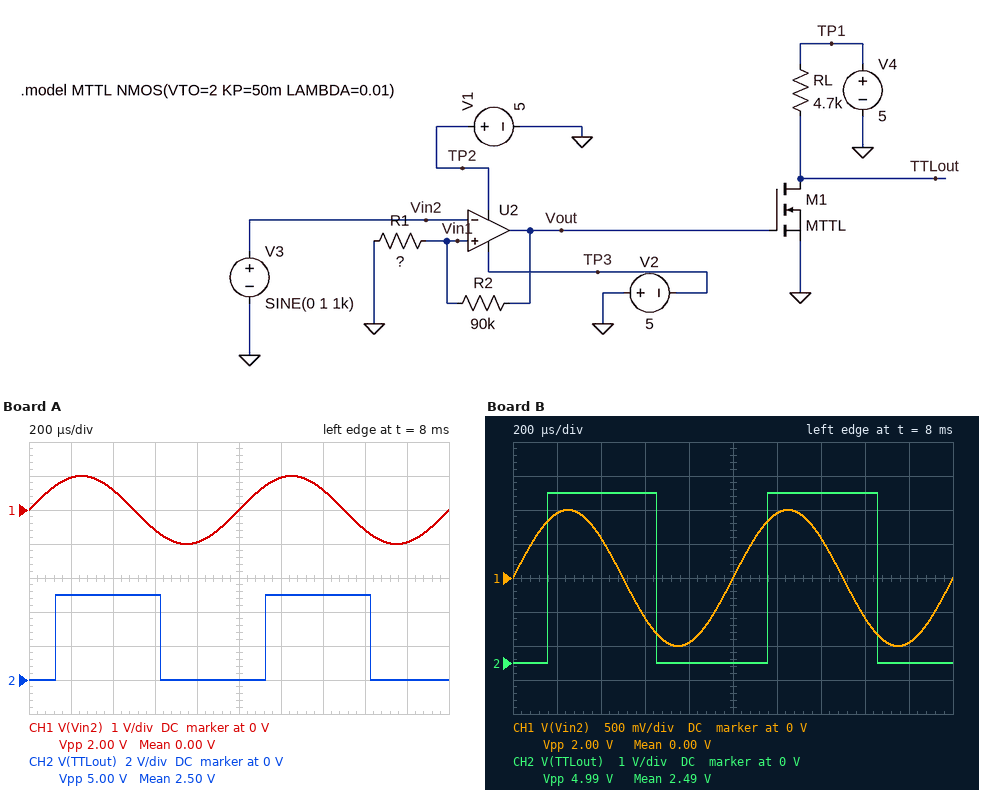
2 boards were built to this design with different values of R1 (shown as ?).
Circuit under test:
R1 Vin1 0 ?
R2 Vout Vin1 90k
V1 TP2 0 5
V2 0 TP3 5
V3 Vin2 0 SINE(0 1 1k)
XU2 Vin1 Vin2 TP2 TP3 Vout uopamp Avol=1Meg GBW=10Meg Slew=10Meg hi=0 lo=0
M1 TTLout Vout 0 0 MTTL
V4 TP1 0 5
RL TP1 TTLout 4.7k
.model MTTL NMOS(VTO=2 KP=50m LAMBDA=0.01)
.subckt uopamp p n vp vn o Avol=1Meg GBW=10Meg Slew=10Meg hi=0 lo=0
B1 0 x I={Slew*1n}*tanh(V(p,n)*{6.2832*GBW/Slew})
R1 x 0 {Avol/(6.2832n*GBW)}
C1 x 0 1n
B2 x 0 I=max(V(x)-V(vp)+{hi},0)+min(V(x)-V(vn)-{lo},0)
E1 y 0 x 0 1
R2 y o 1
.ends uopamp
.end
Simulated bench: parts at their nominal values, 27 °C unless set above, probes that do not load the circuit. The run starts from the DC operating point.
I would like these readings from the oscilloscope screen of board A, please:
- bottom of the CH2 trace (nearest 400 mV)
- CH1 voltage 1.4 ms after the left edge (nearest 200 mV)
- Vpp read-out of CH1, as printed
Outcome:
0 V
600 mV
2.00 V
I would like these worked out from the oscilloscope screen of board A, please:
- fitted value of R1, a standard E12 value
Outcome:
15 kΩ
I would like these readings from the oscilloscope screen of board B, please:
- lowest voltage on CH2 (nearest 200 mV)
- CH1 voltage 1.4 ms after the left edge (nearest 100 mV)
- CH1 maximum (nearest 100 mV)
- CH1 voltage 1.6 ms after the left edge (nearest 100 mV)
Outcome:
0 V
600 mV
1.0 V
-600 mV
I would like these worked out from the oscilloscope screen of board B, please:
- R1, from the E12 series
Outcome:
18 kΩ
